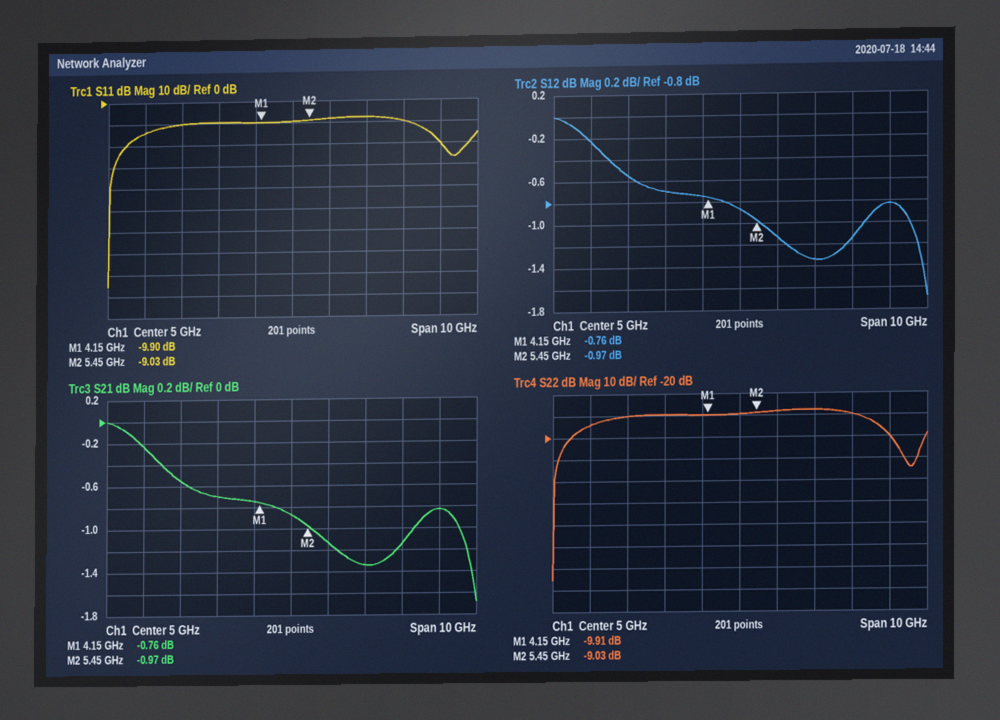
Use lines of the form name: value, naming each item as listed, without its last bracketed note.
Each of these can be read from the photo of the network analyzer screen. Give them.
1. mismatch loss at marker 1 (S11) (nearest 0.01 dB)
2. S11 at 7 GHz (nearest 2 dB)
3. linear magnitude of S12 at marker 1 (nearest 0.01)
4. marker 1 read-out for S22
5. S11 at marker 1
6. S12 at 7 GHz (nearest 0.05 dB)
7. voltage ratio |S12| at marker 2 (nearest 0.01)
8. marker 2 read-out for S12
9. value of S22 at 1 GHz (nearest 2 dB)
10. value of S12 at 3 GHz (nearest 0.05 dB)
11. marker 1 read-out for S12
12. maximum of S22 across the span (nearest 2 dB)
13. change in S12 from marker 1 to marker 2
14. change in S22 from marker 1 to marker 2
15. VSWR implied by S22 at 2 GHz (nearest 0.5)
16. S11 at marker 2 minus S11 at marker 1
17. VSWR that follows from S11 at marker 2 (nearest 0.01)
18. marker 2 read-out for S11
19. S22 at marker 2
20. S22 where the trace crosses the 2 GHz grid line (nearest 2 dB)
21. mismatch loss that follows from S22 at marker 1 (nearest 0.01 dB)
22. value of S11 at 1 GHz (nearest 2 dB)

mismatch loss at marker 1 (S11): 0.47 dB
S11 at 7 GHz: -8 dB
linear magnitude of S12 at marker 1: 0.92
marker 1 read-out for S22: -9.91 dB
S11 at marker 1: -9.90 dB
S12 at 7 GHz: -1.35 dB
voltage ratio |S12| at marker 2: 0.89
marker 2 read-out for S12: -0.97 dB
value of S22 at 1 GHz: -14 dB
value of S12 at 3 GHz: -0.70 dB
marker 1 read-out for S12: -0.76 dB
maximum of S22 across the span: -8 dB
change in S12 from marker 1 to marker 2: -0.21 dB
change in S22 from marker 1 to marker 2: 0.88 dB
VSWR implied by S22 at 2 GHz: 2.0
S11 at marker 2 minus S11 at marker 1: 0.87 dB
VSWR that follows from S11 at marker 2: 2.09
marker 2 read-out for S11: -9.03 dB
S22 at marker 2: -9.03 dB
S22 where the trace crosses the 2 GHz grid line: -10 dB
mismatch loss that follows from S22 at marker 1: 0.47 dB
value of S11 at 1 GHz: -14 dB
